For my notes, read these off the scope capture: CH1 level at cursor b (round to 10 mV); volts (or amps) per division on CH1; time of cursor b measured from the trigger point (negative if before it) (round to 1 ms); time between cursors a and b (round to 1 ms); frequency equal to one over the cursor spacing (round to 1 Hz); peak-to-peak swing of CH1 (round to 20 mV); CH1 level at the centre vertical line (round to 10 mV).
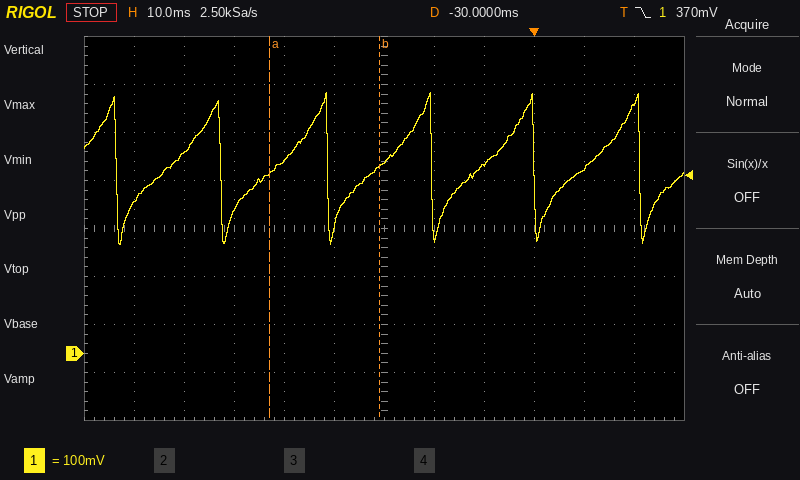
390 mV
100 mV
-31 ms
22 ms
45 Hz
320 mV
400 mV
